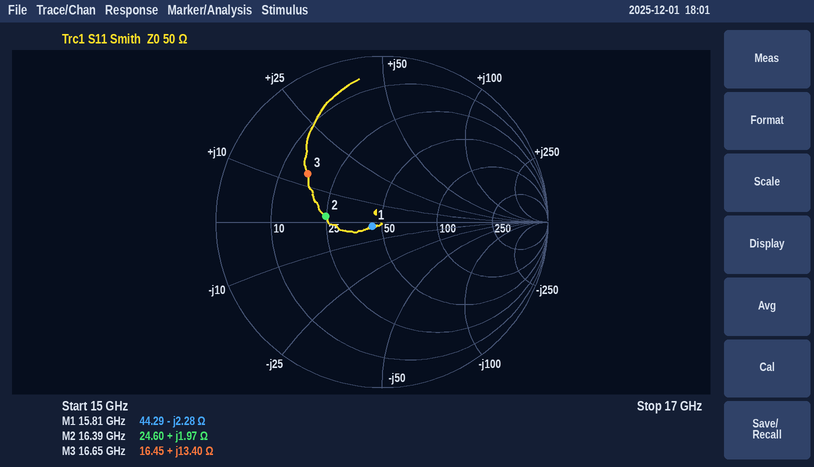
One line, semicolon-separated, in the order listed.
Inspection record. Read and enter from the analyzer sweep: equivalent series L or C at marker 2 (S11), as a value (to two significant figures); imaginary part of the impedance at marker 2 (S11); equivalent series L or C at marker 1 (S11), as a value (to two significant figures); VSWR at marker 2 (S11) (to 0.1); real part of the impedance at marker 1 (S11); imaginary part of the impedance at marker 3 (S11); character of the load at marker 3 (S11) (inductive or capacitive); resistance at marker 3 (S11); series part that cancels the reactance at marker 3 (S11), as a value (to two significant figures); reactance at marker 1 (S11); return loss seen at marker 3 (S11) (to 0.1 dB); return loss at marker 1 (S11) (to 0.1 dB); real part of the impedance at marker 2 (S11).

19 pH; +1.97 Ω; 4.4 pF; 2.0; 44.29 Ω; +13.40 Ω; inductive; 16.45 Ω; 710 fF; -2.28 Ω; 5.5 dB; 23.7 dB; 24.60 Ω
